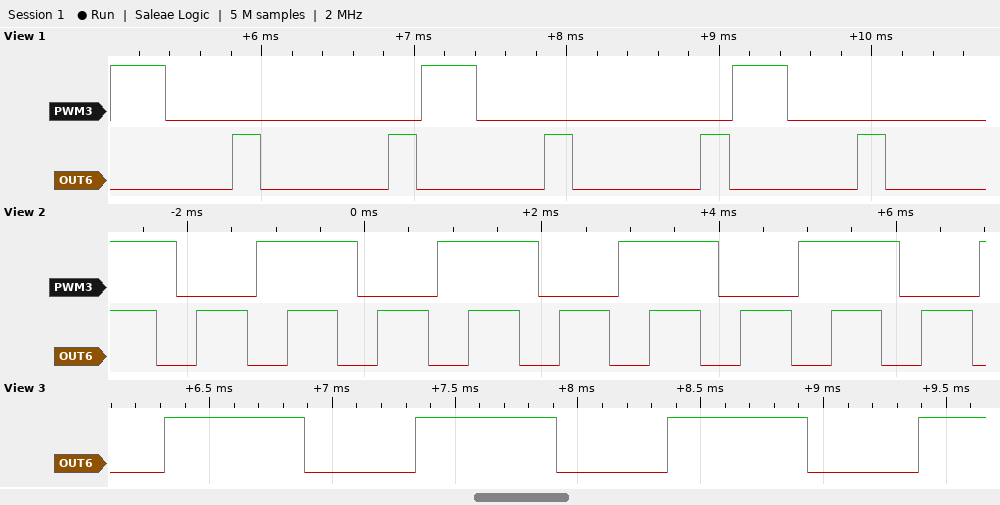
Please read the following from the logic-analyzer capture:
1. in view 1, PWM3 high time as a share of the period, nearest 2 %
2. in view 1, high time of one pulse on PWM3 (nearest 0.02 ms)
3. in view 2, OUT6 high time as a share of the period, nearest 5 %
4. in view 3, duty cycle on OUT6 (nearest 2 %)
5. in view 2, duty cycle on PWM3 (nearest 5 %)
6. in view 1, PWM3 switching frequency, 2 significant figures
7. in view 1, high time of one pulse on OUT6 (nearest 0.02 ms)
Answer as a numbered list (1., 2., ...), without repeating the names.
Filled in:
1. 18 %
2. 0.36 ms
3. 55 %
4. 56 %
5. 55 %
6. 490 Hz
7. 0.18 ms
